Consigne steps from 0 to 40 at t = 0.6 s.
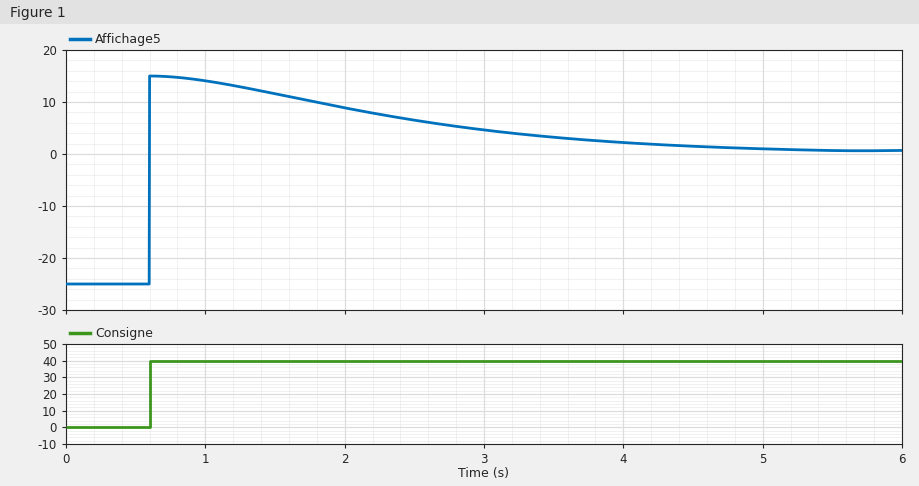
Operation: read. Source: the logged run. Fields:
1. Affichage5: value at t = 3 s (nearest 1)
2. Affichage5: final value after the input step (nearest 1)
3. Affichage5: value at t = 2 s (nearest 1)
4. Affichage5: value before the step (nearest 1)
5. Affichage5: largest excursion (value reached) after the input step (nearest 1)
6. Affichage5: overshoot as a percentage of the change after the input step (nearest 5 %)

5
1
9
-25
15
55 %
